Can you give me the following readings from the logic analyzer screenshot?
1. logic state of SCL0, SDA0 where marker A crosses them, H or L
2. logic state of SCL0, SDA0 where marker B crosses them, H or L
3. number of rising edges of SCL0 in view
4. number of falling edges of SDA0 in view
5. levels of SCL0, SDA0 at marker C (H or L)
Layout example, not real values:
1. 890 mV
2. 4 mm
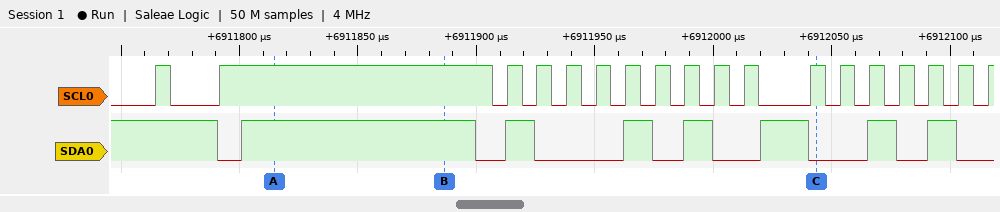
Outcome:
1. SCL0=H, SDA0=H
2. SCL0=H, SDA0=H
3. 18
4. 8
5. SCL0=H, SDA0=L
